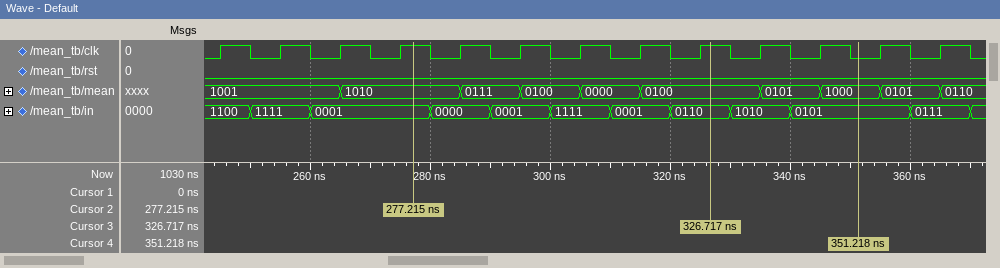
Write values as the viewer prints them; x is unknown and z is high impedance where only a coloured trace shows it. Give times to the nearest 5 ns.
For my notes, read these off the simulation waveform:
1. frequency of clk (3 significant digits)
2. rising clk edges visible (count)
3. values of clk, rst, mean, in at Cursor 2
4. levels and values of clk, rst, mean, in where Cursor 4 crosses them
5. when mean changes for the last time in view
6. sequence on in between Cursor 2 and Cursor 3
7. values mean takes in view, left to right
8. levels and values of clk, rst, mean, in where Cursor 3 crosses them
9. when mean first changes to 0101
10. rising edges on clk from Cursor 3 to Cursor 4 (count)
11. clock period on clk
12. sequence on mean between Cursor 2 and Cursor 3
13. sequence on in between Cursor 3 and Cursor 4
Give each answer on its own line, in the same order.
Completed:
100 MHz
13
clk=1, rst=0, mean=1010, in=0001
clk=0, rst=0, mean=1000, in=0101
365 ns
0001, 0000, 0001, 1111, 0001, 0110
1001, 1010, 0111, 0100, 0000, 0100, 0101, 1000, 0101, 0110
clk=1, rst=0, mean=0100, in=0110
335 ns
2
10 ns
1010, 0111, 0100, 0000, 0100
0110, 1010, 0101
